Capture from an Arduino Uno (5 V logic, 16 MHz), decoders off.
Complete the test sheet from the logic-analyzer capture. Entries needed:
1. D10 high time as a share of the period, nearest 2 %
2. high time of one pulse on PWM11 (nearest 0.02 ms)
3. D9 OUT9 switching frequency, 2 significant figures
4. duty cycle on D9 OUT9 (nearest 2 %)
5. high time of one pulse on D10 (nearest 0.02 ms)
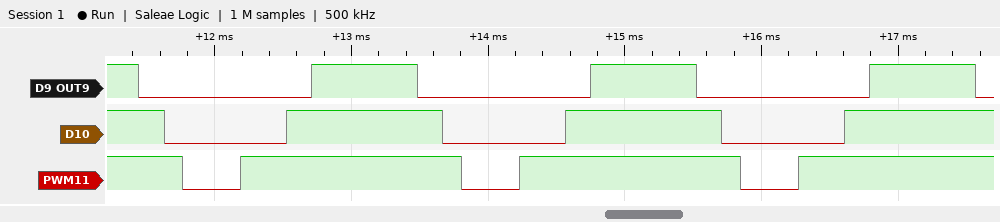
56 %
1.62 ms
490 Hz
38 %
1.14 ms
